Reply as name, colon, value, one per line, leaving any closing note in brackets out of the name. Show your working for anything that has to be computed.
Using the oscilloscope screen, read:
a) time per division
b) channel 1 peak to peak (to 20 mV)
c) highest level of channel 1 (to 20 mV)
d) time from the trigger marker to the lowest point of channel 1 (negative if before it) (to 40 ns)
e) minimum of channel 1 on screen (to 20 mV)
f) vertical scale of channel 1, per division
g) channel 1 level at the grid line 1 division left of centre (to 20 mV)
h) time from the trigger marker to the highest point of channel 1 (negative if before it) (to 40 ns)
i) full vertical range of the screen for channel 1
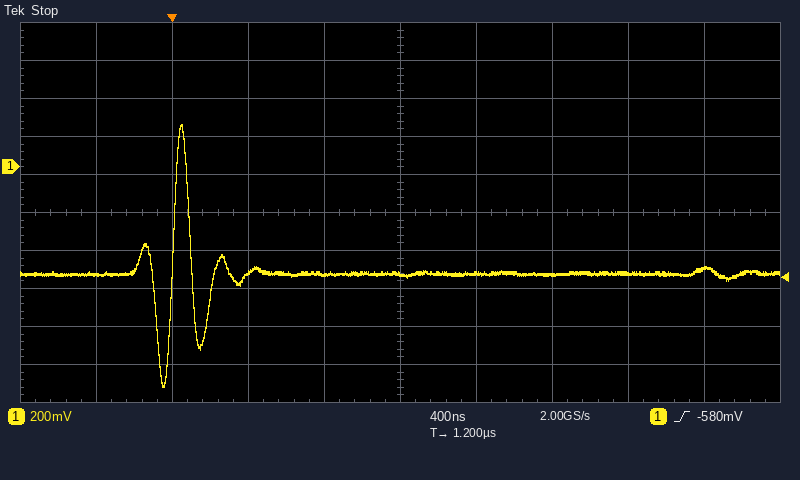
time per division: 400 ns
channel 1 peak to peak: 220 mV − (-1.16 V) = 1.38 V
highest level of channel 1: 220 mV
time from the trigger marker to the lowest point of channel 1 (negative if before it): -40 ns
minimum of channel 1 on screen: -1.16 V
vertical scale of channel 1, per division: 200 mV
channel 1 level at the grid line 1 division left of centre: -560 mV
time from the trigger marker to the highest point of channel 1 (negative if before it): +40 ns
full vertical range of the screen for channel 1: 2 V
